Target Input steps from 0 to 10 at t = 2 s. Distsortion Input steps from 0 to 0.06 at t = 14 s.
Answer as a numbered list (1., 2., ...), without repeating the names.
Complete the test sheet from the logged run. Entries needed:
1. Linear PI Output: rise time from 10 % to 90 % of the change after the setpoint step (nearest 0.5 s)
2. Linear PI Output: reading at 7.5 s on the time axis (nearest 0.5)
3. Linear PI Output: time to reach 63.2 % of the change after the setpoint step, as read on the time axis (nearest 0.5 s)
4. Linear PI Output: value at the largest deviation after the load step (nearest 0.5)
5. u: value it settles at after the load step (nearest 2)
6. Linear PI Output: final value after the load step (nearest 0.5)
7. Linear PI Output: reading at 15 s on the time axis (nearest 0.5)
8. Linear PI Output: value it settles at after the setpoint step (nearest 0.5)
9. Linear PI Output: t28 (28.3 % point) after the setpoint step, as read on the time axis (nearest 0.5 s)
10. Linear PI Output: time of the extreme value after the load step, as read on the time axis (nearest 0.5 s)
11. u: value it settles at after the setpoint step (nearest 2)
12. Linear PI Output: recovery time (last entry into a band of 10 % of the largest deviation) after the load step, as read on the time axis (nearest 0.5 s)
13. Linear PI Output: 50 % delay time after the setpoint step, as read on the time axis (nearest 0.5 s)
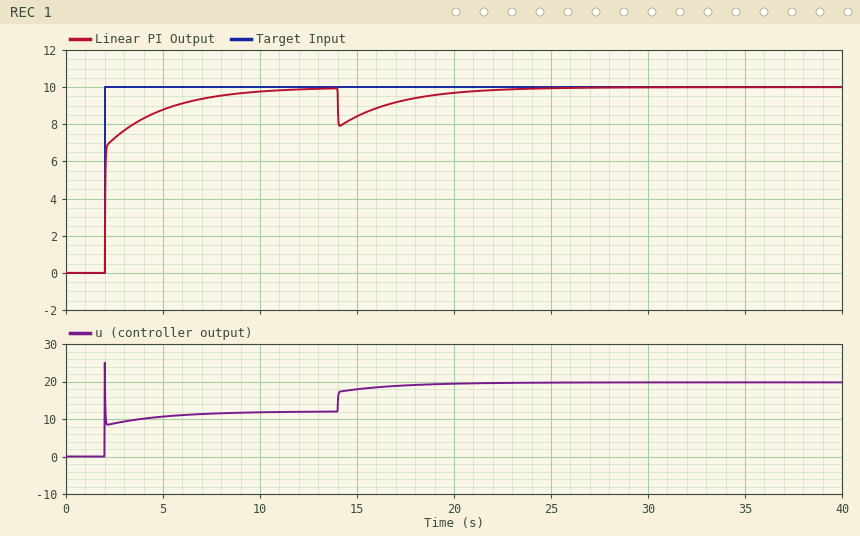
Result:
1. 3.5 s
2. 9.5
3. 2.0 s
4. 8.0
5. 20
6. 10.0
7. 8.5
8. 10.0
9. 2.0 s
10. 14.0 s
11. 12
12. 21.5 s
13. 2.0 s
